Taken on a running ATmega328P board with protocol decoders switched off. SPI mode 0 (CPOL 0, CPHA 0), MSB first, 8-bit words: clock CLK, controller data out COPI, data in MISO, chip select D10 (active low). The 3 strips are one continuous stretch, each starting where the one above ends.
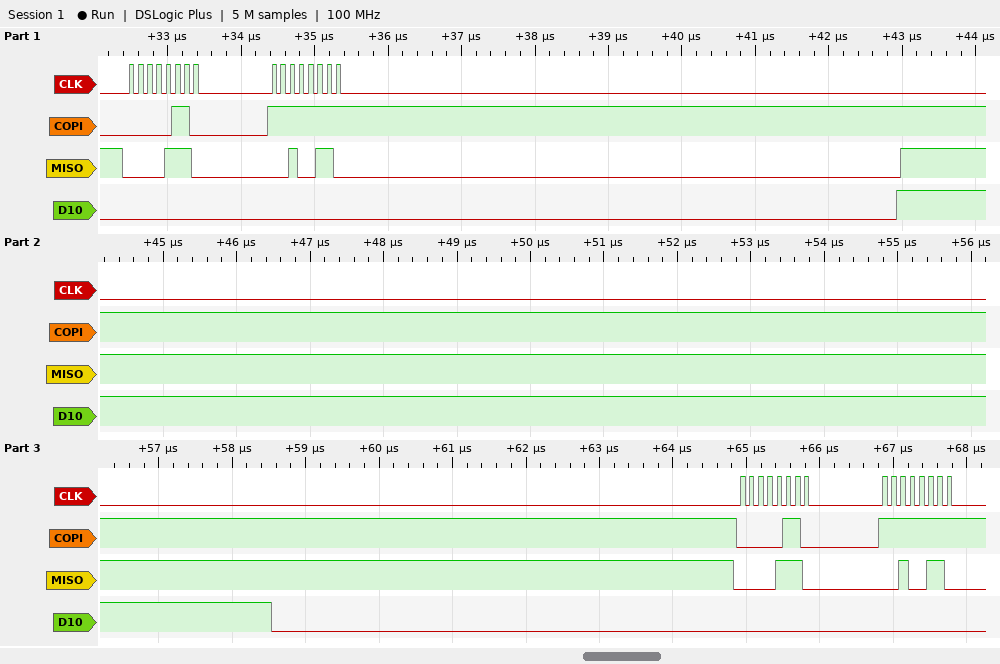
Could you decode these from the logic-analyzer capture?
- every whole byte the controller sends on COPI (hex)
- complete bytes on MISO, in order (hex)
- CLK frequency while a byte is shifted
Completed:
06 FF 06 FF
0E 26 0E 26
8 MHz
